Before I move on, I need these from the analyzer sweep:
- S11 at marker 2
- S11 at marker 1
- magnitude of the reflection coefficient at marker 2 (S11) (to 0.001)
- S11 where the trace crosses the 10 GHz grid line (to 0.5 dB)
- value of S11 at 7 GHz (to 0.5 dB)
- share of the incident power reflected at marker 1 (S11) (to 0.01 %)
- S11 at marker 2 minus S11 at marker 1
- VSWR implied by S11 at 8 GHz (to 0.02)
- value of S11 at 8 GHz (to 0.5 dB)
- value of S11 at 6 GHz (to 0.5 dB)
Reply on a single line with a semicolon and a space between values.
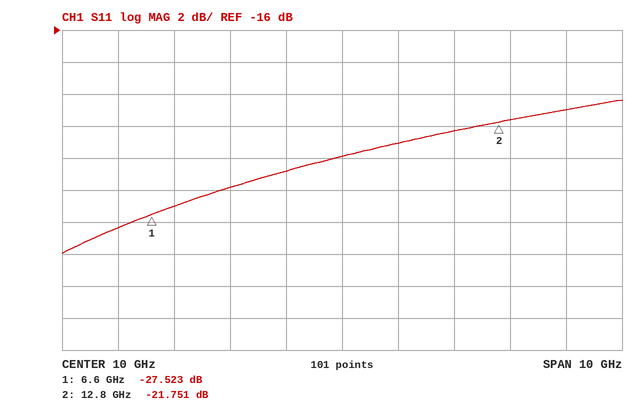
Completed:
-21.751 dB; -27.523 dB; 0.082; -24.0 dB; -27.0 dB; 0.18 %; 5.772 dB; 1.10; -26.0 dB; -28.5 dB
